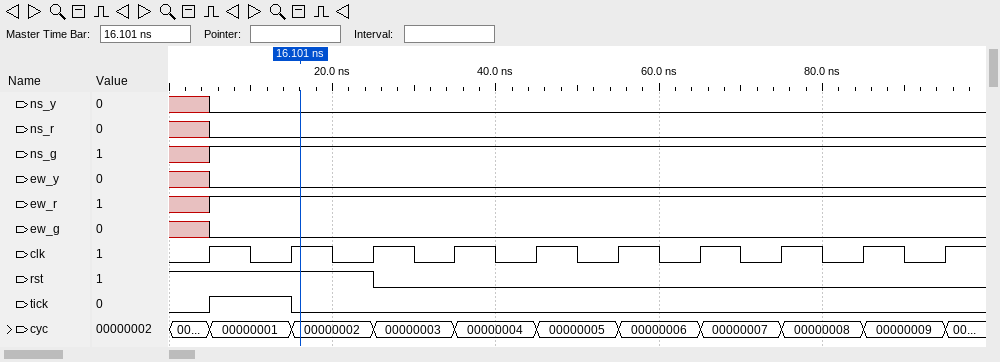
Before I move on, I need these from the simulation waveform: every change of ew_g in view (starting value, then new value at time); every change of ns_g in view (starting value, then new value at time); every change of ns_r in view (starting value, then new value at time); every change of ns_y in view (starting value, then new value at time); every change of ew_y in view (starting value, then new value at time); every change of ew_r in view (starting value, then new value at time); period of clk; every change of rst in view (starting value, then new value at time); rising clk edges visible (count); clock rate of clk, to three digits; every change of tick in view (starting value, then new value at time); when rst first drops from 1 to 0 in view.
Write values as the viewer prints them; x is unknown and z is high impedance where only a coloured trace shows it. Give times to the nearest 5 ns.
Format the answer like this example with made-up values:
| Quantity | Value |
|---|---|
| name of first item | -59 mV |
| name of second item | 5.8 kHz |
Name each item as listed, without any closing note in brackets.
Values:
| Quantity | Value |
|---|---|
| every change of ew_g in view | x, 0 at 5 ns |
| every change of ns_g in view | x, 1 at 5 ns |
| every change of ns_r in view | x, 0 at 5 ns |
| every change of ns_y in view | x, 0 at 5 ns |
| every change of ew_y in view | x, 0 at 5 ns |
| every change of ew_r in view | x, 1 at 5 ns |
| period of clk | 10 ns |
| every change of rst in view | 1, 0 at 25 ns |
| rising clk edges visible | 10 |
| clock rate of clk, to three digits | 100 MHz |
| every change of tick in view | 0, 1 at 5 ns, 0 at 15 ns |
| when rst first drops from 1 to 0 in view | 25 ns |
